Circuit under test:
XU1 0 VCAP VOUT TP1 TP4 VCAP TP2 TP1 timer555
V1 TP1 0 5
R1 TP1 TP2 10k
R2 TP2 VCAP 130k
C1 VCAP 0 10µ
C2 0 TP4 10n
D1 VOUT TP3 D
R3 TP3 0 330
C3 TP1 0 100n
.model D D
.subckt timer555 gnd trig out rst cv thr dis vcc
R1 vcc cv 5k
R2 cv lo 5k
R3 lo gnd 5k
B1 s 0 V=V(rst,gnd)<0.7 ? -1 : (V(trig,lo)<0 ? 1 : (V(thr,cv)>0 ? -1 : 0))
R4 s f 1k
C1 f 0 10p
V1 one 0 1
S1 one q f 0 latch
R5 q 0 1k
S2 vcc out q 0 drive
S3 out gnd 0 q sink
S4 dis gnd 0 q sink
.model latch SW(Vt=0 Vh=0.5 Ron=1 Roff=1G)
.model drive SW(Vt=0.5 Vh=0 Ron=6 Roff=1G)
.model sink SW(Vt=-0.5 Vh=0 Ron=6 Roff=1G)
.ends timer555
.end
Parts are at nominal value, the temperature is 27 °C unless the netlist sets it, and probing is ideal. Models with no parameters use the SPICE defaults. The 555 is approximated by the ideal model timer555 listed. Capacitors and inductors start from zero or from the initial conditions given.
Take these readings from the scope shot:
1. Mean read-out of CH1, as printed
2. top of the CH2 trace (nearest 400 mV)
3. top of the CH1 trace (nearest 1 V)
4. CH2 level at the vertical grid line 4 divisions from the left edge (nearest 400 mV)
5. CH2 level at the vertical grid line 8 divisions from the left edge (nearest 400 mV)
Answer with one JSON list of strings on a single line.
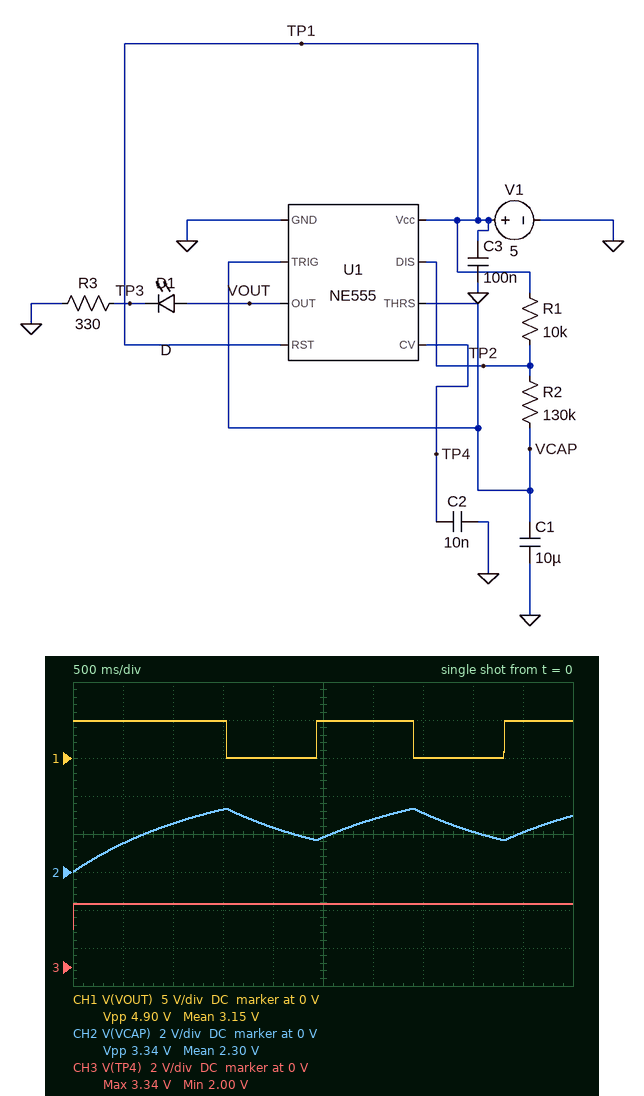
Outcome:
["3.15 V", "3.2 V", "5 V", "2.4 V", "2.0 V"]
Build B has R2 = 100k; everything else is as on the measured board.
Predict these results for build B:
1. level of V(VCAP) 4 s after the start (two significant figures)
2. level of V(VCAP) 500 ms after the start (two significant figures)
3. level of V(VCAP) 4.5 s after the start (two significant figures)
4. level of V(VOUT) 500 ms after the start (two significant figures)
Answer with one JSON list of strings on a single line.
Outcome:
["3.1 V", "1.8 V", "2.3 V", "4.9 V"]
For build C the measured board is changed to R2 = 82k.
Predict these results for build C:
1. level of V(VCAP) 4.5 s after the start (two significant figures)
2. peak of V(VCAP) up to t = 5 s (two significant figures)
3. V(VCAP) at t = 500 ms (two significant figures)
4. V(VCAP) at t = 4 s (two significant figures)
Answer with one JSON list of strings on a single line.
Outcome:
["3.1 V", "3.3 V", "2.1 V", "1.7 V"]
